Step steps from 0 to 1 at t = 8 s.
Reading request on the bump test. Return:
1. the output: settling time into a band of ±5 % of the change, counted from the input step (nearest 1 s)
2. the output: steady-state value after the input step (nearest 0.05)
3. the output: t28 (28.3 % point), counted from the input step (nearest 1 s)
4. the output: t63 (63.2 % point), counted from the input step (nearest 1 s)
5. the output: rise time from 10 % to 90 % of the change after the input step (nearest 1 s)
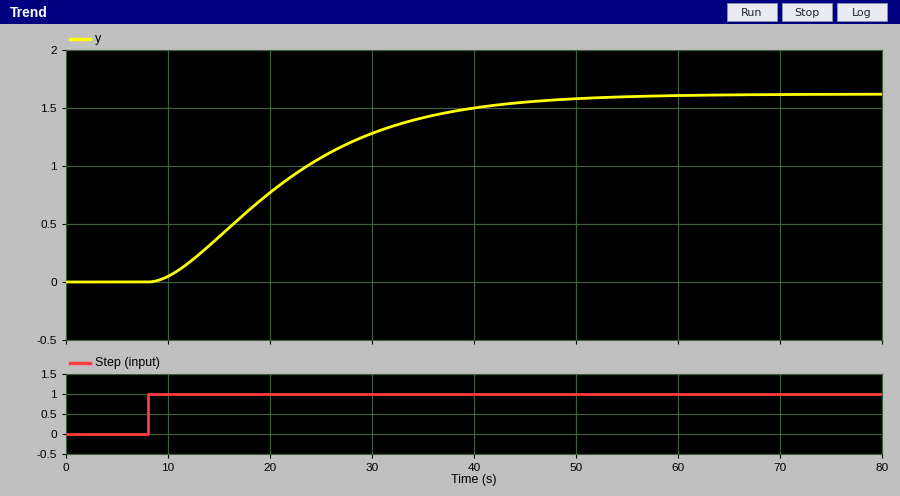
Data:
36 s
1.60
8 s
16 s
25 s
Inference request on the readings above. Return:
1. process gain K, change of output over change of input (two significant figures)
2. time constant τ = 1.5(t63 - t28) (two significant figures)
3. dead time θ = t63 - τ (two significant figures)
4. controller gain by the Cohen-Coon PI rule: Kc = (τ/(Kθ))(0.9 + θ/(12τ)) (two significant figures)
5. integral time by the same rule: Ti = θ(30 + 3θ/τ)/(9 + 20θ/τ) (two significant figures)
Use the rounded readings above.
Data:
1.6
12 s
4.0 s
1.7
7.9 s
